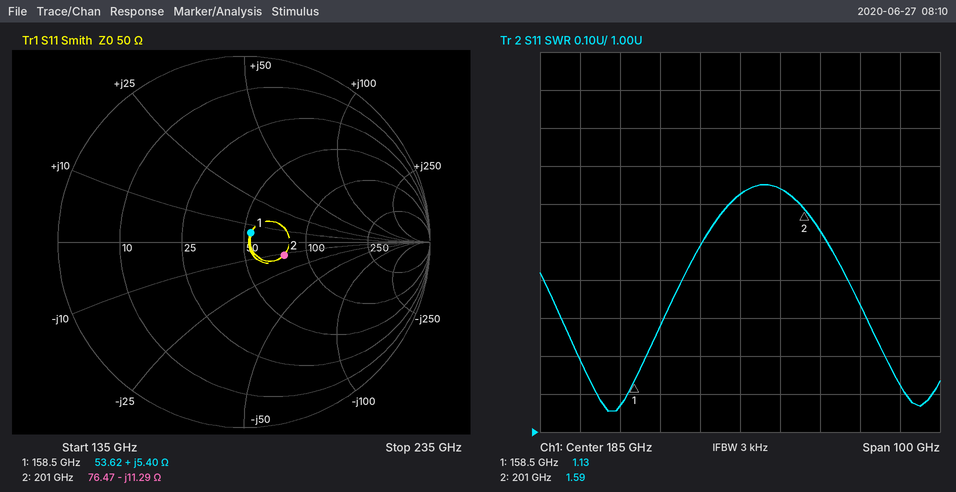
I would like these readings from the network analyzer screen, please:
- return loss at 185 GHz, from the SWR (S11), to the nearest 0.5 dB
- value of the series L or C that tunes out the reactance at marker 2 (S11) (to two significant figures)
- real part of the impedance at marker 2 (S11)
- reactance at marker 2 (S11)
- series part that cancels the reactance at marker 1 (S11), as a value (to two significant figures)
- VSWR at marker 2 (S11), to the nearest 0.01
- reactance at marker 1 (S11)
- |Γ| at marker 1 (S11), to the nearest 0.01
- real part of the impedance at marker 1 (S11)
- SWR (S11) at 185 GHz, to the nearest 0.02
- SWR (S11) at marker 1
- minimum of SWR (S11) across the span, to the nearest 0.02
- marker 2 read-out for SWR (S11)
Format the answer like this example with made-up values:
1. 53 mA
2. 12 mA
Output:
1. 12.5 dB
2. 8.9 pH
3. 76.47 Ω
4. -11.29 Ω
5. 190 fF
6. 1.59
7. +5.40 Ω
8. 0.06
9. 53.62 Ω
10. 1.62
11. 1.13
12. 1.06
13. 1.59
